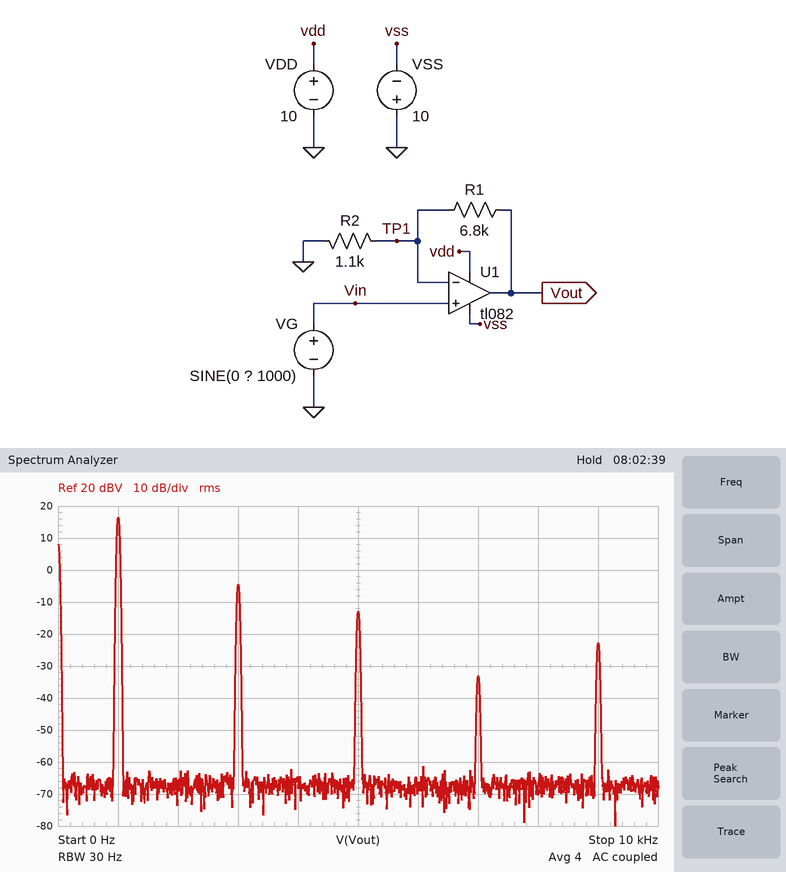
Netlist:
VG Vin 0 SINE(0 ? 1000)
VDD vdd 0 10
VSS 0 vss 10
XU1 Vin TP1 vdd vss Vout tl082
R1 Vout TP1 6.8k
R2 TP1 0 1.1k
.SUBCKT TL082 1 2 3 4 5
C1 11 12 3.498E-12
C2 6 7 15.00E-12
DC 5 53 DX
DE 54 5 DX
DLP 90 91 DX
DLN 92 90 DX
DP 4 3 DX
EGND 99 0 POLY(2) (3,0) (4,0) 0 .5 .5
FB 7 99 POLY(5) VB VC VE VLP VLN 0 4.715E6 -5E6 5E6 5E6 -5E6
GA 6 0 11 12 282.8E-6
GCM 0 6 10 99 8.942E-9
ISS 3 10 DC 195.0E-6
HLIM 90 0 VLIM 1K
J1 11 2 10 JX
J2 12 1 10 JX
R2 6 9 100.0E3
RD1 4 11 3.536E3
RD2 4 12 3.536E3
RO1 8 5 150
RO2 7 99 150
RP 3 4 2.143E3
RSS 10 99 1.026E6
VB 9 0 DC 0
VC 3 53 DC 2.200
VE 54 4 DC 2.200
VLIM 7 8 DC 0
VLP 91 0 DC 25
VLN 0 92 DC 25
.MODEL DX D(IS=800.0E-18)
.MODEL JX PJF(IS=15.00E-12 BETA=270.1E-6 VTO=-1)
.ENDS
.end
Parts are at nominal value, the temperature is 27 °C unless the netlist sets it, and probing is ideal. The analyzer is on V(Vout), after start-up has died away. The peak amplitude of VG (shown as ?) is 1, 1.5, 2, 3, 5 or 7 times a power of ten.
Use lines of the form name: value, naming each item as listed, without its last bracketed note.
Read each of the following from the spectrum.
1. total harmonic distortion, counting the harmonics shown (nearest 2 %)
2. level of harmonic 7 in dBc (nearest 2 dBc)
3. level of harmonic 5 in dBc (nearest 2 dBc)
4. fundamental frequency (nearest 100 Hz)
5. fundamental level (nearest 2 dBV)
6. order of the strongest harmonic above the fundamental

total harmonic distortion, counting the harmonics shown: 10 %
level of harmonic 7 in dBc: -50 dBc
level of harmonic 5 in dBc: -30 dBc
fundamental frequency: 1.0 kHz
fundamental level: 16 dBV
order of the strongest harmonic above the fundamental: 3
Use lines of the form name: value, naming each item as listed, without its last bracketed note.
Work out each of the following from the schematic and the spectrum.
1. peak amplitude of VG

peak amplitude of VG: 1.5 V
